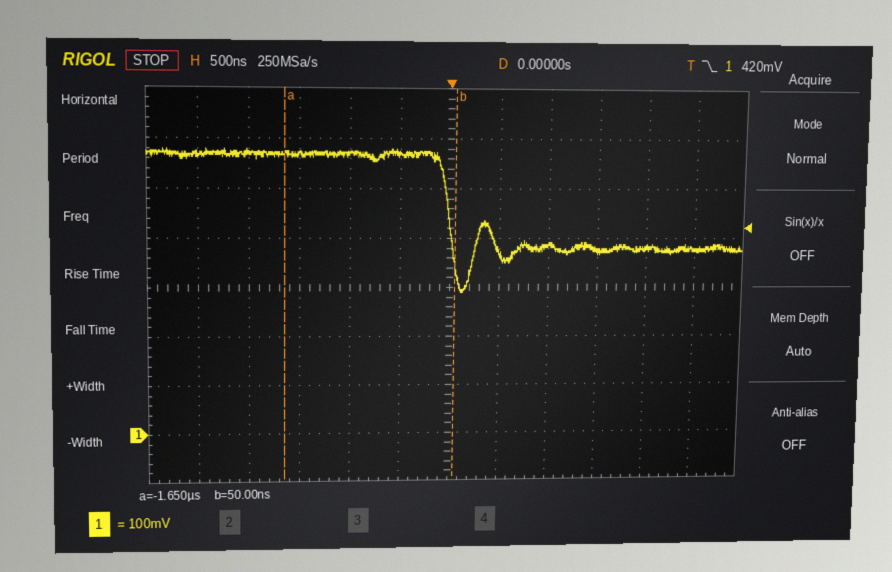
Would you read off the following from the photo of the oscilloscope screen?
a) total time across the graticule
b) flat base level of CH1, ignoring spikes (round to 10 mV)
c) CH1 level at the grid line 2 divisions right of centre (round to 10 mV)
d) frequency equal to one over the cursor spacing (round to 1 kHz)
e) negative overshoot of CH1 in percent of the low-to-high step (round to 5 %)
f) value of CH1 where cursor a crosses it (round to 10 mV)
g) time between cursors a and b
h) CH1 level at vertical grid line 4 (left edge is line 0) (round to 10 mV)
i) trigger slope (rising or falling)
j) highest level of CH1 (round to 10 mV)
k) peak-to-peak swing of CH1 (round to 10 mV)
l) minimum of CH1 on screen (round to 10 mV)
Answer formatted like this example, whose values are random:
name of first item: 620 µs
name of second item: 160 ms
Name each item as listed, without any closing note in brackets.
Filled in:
total time across the graticule: 6 µs
flat base level of CH1, ignoring spikes: 380 mV
CH1 level at the grid line 2 divisions right of centre: 390 mV
frequency equal to one over the cursor spacing: 588 kHz
negative overshoot of CH1 in percent of the low-to-high step: 45 %
value of CH1 where cursor a crosses it: 570 mV
time between cursors a and b: 1.70 µs
CH1 level at vertical grid line 4 (left edge is line 0): 570 mV
trigger slope: falling
highest level of CH1: 580 mV
peak-to-peak swing of CH1: 290 mV
minimum of CH1 on screen: 290 mV
